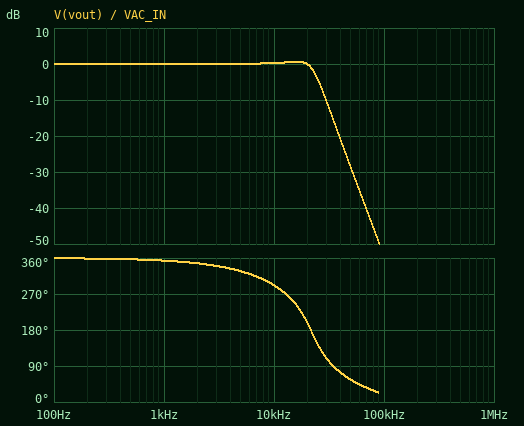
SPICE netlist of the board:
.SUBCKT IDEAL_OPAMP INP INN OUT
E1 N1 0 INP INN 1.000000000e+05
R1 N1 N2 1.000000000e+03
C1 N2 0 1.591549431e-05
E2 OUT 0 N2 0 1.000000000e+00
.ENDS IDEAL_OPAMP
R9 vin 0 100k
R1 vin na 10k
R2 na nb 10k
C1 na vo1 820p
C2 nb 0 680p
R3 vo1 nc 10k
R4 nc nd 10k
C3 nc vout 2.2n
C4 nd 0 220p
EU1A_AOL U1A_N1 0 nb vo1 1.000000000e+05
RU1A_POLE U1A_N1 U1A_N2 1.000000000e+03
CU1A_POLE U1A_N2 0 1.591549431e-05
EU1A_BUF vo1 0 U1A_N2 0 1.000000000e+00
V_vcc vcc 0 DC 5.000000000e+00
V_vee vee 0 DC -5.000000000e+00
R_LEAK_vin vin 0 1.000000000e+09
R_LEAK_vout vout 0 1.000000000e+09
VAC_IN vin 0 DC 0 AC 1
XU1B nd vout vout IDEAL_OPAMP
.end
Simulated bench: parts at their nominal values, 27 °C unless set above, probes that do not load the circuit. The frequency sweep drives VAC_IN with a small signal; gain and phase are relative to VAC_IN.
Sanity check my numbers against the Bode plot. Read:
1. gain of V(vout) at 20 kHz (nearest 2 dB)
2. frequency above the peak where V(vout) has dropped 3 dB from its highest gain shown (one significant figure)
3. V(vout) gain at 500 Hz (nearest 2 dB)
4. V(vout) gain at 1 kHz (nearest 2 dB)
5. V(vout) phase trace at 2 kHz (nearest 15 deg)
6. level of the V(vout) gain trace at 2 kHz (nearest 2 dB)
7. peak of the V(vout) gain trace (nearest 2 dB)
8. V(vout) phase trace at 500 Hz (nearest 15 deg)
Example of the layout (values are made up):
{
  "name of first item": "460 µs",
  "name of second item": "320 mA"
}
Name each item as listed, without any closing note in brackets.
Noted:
{
  "gain of V(vout) at 20 kHz": "0 dB",
  "frequency above the peak where V(vout) has dropped 3 dB from its highest gain shown": "20 kHz",
  "V(vout) gain at 500 Hz": "0 dB",
  "V(vout) gain at 1 kHz": "0 dB",
  "V(vout) phase trace at 2 kHz": "345 deg",
  "level of the V(vout) gain trace at 2 kHz": "0 dB",
  "peak of the V(vout) gain trace": "0 dB",
  "V(vout) phase trace at 500 Hz": "360 deg"
}
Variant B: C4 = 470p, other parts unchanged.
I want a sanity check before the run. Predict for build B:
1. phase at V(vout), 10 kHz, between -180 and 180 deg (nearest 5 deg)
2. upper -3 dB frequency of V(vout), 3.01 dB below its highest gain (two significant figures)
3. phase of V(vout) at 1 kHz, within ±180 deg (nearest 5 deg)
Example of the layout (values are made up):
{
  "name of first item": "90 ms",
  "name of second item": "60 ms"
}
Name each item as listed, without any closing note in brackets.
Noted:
{
  "phase at V(vout), 10 kHz, between -180 and 180 deg": "-95 deg",
  "upper -3 dB frequency of V(vout), 3.01 dB below its highest gain": "16 kHz",
  "phase of V(vout) at 1 kHz, within ±180 deg": "-10 deg"
}
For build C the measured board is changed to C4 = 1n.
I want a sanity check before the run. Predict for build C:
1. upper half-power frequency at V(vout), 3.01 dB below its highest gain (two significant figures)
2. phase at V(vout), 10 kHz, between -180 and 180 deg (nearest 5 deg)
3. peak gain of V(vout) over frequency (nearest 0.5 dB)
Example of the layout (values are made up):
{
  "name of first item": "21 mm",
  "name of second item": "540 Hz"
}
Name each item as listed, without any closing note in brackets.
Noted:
{
  "upper half-power frequency at V(vout), 3.01 dB below its highest gain": "9.7 kHz",
  "phase at V(vout), 10 kHz, between -180 and 180 deg": "-135 deg",
  "peak gain of V(vout) over frequency": "0 dB"
}
